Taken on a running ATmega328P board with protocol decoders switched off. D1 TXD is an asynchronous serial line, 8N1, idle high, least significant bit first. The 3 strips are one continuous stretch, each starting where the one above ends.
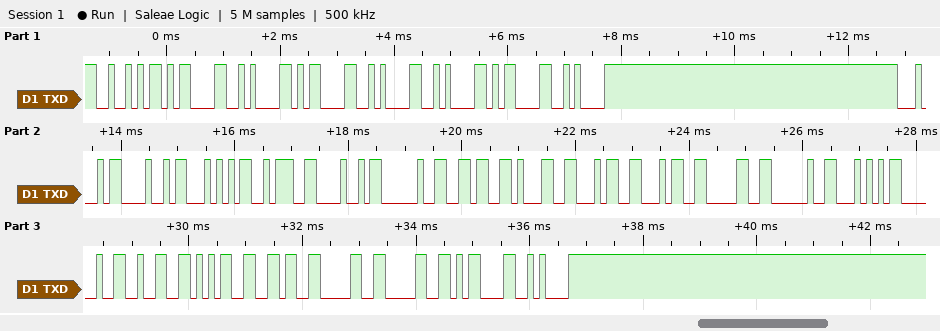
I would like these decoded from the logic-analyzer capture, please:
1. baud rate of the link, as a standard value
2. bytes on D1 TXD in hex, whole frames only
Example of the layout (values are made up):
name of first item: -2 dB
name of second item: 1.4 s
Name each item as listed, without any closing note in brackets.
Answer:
baud rate of the link, as a standard value: 9600 baud
bytes on D1 TXD in hex, whole frames only: 52 0D 0A 0D 0A 0A 0D 0A 44 48 54 3A 48 20 36 31 34 34 30 20 54 20 32 35 36 30 30 0D 0A
